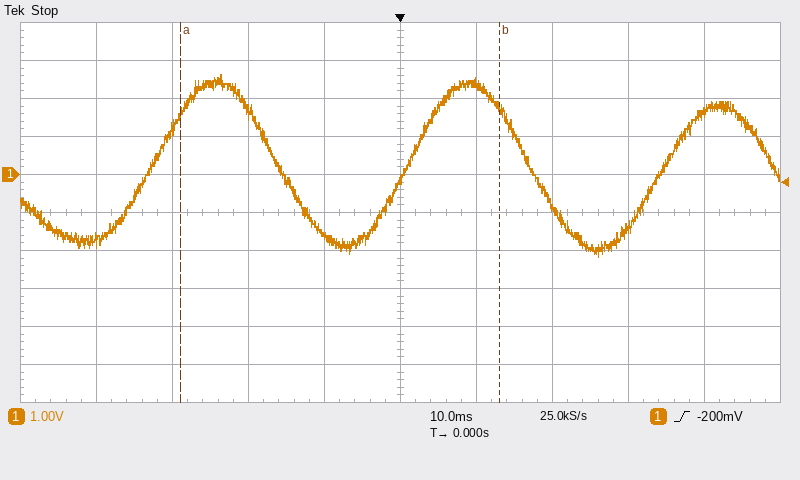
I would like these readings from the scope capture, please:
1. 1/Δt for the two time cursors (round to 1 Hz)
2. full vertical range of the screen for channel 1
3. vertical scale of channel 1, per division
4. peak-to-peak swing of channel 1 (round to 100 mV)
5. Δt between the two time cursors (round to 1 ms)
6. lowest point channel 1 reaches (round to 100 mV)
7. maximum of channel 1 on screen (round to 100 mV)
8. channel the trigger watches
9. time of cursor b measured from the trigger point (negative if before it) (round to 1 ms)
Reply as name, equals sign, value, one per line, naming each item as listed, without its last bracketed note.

1/Δt for the two time cursors = 24 Hz
full vertical range of the screen for channel 1 = 10 V
vertical scale of channel 1, per division = 1 V
peak-to-peak swing of channel 1 = 4.8 V
Δt between the two time cursors = 42 ms
lowest point channel 1 reaches = -2.2 V
maximum of channel 1 on screen = 2.6 V
channel the trigger watches = channel 1
time of cursor b measured from the trigger point (negative if before it) = +13 ms
